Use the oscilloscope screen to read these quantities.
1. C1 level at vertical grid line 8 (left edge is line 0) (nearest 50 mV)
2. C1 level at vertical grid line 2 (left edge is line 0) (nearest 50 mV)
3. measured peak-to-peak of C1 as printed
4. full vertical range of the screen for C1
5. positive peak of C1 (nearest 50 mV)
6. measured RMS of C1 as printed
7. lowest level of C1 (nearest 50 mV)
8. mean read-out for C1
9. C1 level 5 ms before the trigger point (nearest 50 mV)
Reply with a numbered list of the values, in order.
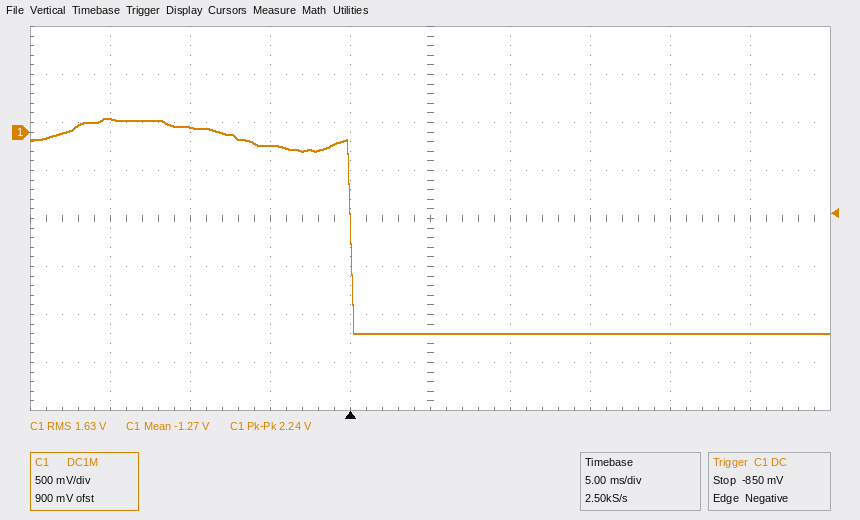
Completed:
1. -2.10 V
2. 50 mV
3. 2.24 V
4. 4 V
5. 150 mV
6. 1.63 V
7. -2.10 V
8. -1.27 V
9. -150 mV
